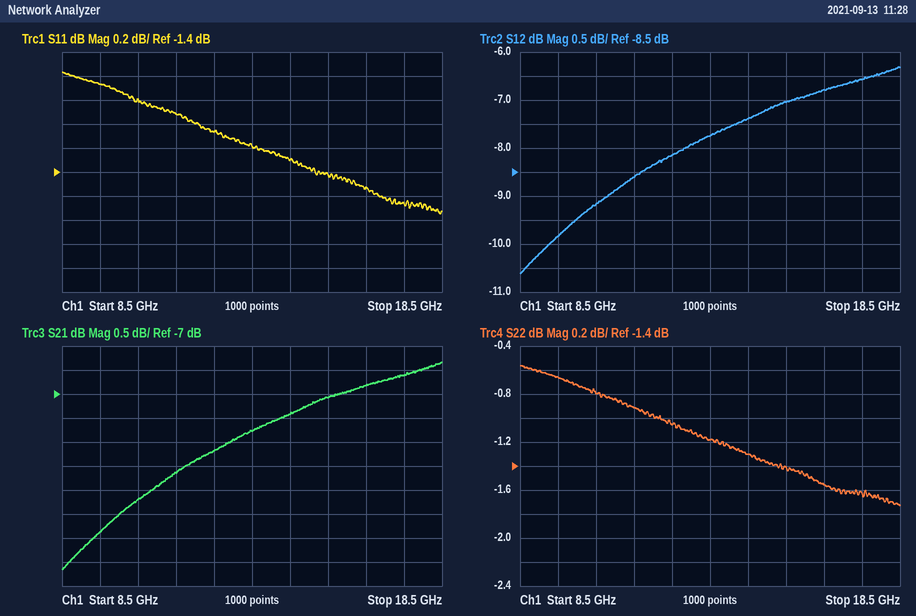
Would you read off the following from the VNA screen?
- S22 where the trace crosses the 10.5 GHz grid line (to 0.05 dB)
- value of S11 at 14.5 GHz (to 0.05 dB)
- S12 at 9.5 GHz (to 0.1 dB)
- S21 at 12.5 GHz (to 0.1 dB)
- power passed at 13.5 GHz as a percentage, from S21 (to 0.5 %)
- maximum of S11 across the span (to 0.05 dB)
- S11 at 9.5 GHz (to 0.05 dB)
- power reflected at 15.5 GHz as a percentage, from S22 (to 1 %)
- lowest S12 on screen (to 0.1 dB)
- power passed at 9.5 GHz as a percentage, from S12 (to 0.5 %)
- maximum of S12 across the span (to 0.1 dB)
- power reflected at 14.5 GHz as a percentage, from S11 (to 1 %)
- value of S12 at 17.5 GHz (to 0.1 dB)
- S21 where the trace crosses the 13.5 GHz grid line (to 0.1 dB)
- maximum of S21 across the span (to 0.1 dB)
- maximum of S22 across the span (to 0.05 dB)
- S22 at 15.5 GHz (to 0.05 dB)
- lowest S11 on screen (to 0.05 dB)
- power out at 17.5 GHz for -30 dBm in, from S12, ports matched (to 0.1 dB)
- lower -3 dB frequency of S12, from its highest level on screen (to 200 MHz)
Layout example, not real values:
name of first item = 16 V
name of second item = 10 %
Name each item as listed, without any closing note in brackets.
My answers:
S22 where the trace crosses the 10.5 GHz grid line = -0.80 dB
value of S11 at 14.5 GHz = -1.30 dB
S12 at 9.5 GHz = -9.8 dB
S21 at 12.5 GHz = -8.2 dB
power passed at 13.5 GHz as a percentage, from S21 = 16.5 %
maximum of S11 across the span = -0.55 dB
S11 at 9.5 GHz = -0.65 dB
power reflected at 15.5 GHz as a percentage, from S22 = 72 %
lowest S12 on screen = -10.6 dB
power passed at 9.5 GHz as a percentage, from S12 = 10.5 %
maximum of S12 across the span = -6.3 dB
power reflected at 14.5 GHz as a percentage, from S11 = 74 %
value of S12 at 17.5 GHz = -6.6 dB
S21 where the trace crosses the 13.5 GHz grid line = -7.8 dB
maximum of S21 across the span = -6.3 dB
maximum of S22 across the span = -0.55 dB
S22 at 15.5 GHz = -1.40 dB
lowest S11 on screen = -1.75 dB
power out at 17.5 GHz for -30 dBm in, from S12, ports matched = -36.6 dBm
lower -3 dB frequency of S12, from its highest level on screen = 10.2 GHz
